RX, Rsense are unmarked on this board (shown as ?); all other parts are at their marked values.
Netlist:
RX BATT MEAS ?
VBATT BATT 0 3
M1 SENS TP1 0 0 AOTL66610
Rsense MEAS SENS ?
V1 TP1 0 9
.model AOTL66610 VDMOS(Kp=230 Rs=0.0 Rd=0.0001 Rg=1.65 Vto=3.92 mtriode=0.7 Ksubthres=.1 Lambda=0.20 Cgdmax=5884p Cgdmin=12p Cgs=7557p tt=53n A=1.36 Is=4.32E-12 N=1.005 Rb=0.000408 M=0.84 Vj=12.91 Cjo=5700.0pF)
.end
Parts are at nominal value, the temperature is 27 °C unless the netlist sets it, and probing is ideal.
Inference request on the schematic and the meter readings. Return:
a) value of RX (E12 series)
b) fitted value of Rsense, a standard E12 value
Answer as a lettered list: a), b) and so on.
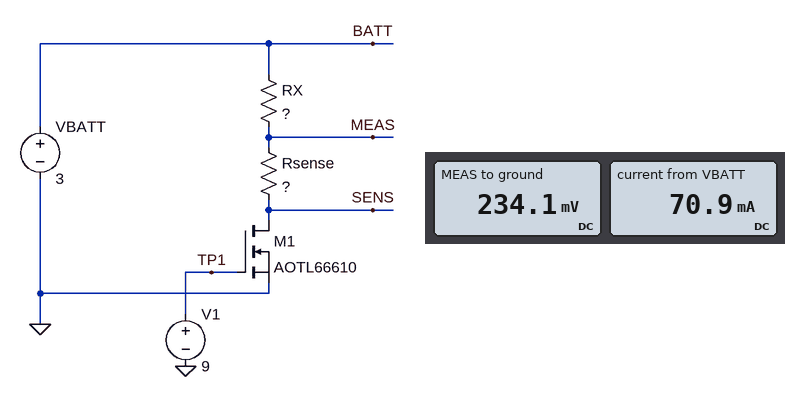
a) 39 Ω
b) 3.3 Ω
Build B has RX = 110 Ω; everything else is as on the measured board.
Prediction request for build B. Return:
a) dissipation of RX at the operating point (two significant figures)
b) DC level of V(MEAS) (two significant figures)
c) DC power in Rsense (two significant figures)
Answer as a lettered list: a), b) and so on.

a) 77 mW
b) 87 mV
c) 2.3 mW
